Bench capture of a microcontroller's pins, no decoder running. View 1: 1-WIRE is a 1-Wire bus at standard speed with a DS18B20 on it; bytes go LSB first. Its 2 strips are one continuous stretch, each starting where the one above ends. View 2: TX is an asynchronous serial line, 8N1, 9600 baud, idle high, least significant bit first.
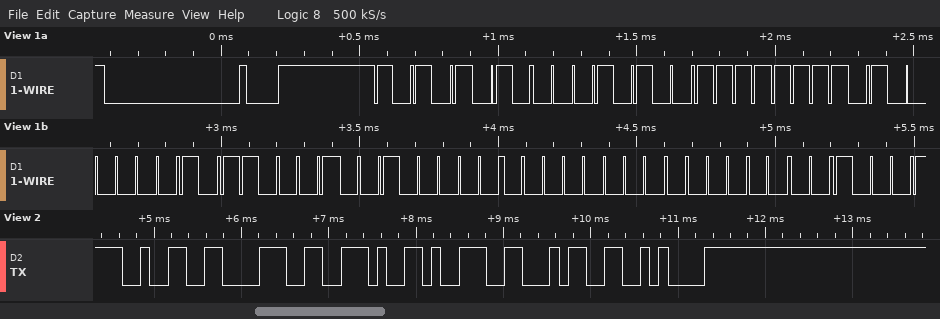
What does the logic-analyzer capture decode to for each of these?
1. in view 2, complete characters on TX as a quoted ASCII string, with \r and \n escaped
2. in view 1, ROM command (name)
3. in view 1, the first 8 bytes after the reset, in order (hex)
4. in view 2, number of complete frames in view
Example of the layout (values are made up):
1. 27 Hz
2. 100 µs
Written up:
1. "28.94\n"
2. Match ROM
3. 55 28 FF 02 8D 04 00 00
4. 6
